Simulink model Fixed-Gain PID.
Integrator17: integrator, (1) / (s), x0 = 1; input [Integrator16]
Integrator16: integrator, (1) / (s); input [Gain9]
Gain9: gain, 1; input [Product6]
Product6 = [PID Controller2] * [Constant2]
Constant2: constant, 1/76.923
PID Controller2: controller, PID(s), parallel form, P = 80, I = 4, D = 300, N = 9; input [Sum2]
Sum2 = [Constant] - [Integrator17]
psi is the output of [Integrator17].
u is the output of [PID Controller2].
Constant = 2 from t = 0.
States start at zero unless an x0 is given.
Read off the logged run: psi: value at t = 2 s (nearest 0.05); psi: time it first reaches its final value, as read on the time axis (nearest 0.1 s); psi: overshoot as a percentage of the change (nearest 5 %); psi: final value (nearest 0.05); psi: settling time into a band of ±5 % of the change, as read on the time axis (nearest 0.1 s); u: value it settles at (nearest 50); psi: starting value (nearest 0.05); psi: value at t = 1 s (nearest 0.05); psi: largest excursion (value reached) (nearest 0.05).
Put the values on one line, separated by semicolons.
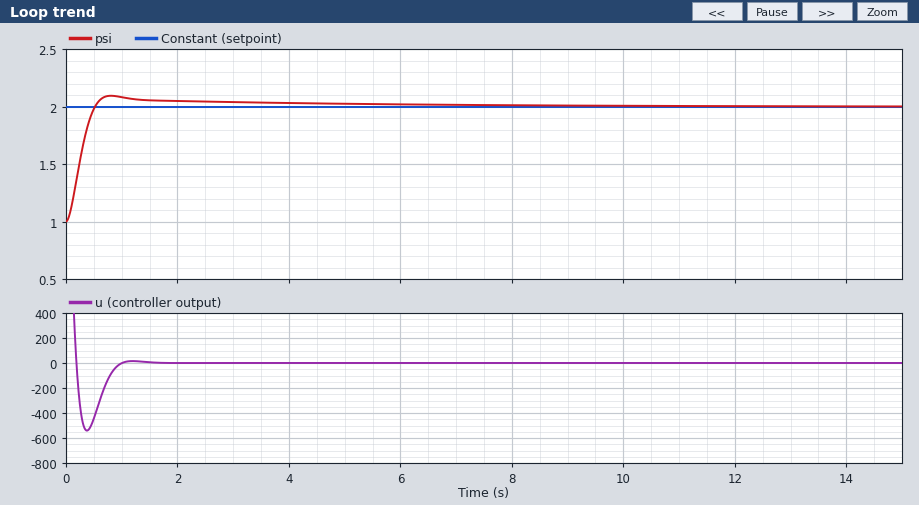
2.05; 0.5 s; 10 %; 2.00; 1.8 s; 0; 1.00; 2.10; 2.10
